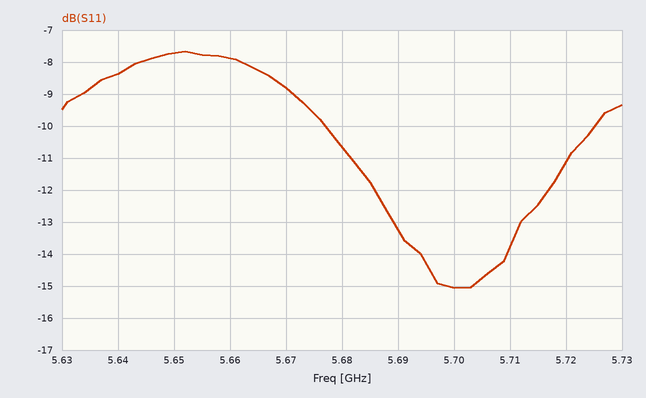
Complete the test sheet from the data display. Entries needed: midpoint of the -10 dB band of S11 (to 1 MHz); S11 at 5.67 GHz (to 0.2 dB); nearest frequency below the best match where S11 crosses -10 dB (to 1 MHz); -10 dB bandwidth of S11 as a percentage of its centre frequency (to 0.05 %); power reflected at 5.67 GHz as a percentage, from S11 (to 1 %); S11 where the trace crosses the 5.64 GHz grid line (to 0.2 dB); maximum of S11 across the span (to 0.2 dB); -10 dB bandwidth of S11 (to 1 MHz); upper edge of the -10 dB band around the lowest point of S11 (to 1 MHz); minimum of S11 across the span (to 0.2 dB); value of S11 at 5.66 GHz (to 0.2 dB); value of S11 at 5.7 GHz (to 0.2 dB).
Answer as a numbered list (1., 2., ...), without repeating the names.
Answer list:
1. 5.701 GHz
2. -8.8 dB
3. 5.677 GHz
4. 0.85 %
5. 13 %
6. -8.4 dB
7. -7.6 dB
8. 48 MHz
9. 5.725 GHz
10. -15.0 dB
11. -7.8 dB
12. -15.0 dB
